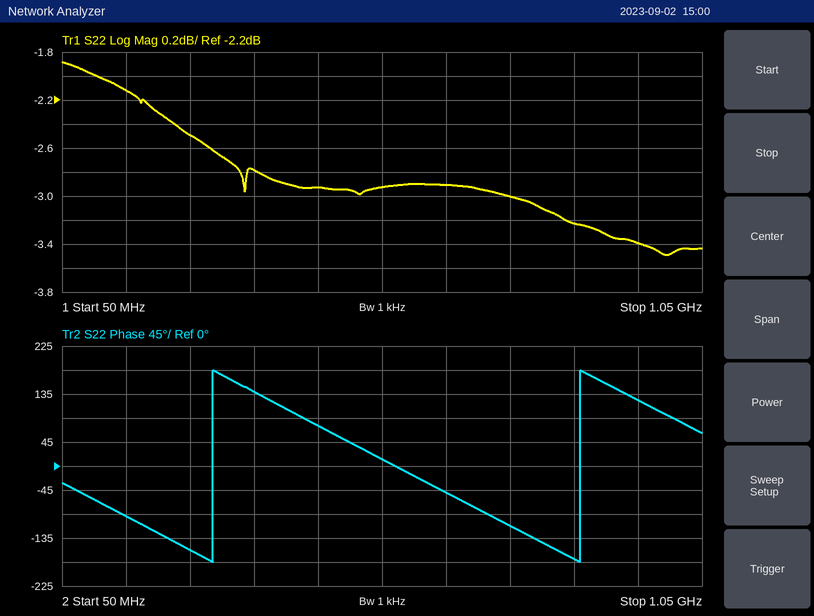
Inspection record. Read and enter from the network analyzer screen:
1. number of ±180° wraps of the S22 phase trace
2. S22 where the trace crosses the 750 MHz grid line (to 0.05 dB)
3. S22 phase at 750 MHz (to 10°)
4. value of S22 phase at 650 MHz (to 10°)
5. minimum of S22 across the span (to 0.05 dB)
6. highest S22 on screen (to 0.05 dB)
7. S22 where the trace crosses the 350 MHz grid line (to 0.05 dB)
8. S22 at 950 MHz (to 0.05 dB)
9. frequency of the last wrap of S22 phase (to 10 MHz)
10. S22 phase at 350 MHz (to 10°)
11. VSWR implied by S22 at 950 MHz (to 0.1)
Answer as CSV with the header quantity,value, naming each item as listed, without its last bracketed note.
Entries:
quantity,value
number of ±180° wraps of the S22 phase trace,2
S22 where the trace crosses the 750 MHz grid line,-3.00 dB
S22 phase at 750 MHz,-110°
value of S22 phase at 650 MHz,-50°
minimum of S22 across the span,-3.50 dB
highest S22 on screen,-1.90 dB
S22 where the trace crosses the 350 MHz grid line,-2.80 dB
S22 at 950 MHz,-3.40 dB
frequency of the last wrap of S22 phase,860 MHz
S22 phase at 350 MHz,140°
VSWR implied by S22 at 950 MHz,5.2
